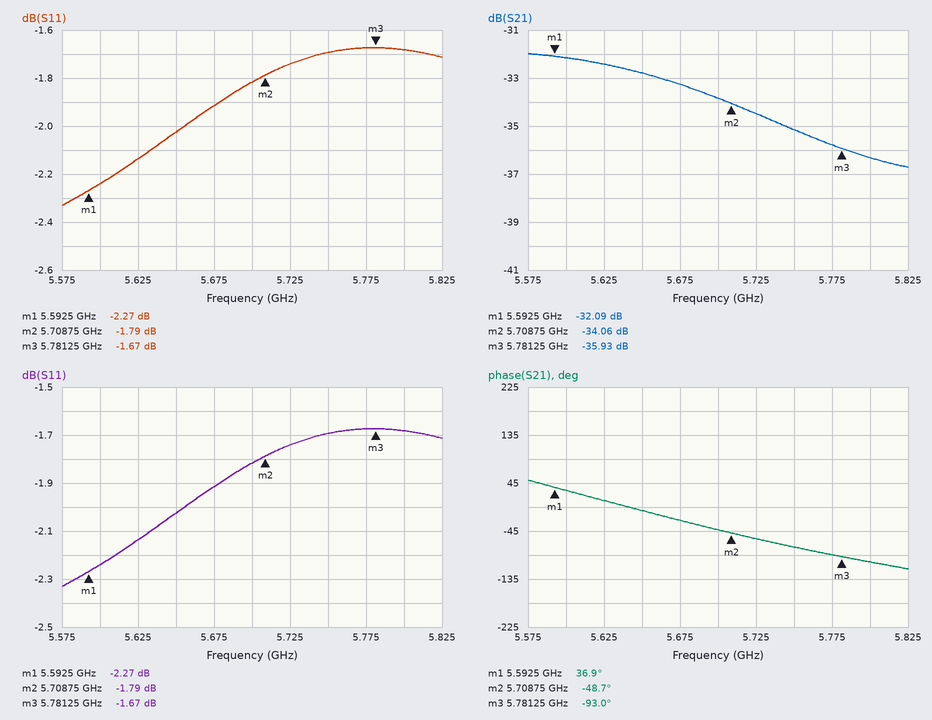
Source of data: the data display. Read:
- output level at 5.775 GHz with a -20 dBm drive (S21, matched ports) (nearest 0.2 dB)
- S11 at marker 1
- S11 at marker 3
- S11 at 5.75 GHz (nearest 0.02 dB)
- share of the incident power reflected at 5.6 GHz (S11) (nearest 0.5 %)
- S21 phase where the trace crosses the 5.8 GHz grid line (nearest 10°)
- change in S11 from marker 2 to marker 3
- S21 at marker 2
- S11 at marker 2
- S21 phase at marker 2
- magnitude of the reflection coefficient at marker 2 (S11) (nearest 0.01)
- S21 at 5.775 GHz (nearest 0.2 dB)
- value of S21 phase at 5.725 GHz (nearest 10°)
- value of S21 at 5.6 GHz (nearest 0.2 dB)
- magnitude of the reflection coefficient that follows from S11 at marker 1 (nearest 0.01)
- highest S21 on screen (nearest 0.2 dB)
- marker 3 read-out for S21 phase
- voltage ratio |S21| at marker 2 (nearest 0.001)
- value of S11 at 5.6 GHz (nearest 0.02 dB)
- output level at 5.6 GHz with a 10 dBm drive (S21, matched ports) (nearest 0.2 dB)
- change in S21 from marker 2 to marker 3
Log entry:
-55.8 dBm
-2.27 dB
-1.67 dB
-1.70 dB
59.5 %
-100°
0.12 dB
-34.06 dB
-1.79 dB
-48.7°
0.81
-35.8 dB
-60°
-32.2 dB
0.77
-32.0 dB
-93.0°
0.020
-2.24 dB
-22.2 dBm
-1.87 dB
